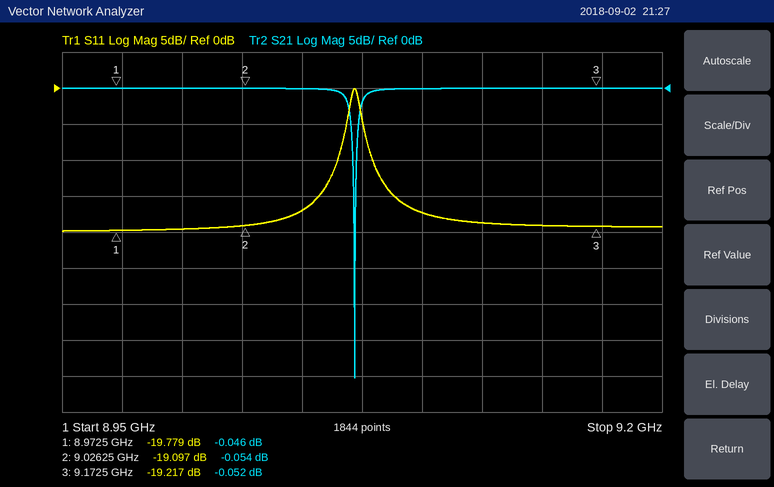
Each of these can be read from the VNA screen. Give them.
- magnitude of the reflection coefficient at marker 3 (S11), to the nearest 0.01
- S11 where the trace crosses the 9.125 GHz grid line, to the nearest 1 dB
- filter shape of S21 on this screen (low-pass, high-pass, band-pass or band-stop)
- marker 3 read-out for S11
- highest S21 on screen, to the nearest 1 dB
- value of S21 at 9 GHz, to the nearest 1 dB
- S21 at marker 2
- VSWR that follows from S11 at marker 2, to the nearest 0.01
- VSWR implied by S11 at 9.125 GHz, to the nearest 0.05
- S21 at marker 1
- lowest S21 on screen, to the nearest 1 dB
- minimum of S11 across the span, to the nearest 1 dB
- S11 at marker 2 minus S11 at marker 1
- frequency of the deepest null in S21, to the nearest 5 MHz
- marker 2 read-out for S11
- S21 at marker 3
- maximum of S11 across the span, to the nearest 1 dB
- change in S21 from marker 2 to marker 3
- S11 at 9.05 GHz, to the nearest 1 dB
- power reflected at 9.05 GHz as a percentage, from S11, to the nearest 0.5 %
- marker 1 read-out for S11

0.11
-19 dB
band-stop
-19.217 dB
0 dB
0 dB
-0.054 dB
1.25
1.25
-0.046 dB
-40 dB
-20 dB
0.682 dB
9.070 GHz
-19.097 dB
-0.052 dB
0 dB
0.002 dB
-17 dB
2.0 %
-19.779 dB
